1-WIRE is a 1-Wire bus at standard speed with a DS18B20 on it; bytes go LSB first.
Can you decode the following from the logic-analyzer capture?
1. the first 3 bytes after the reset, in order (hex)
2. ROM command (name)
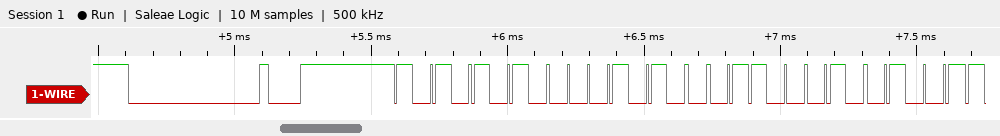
55 28 46
Match ROM
